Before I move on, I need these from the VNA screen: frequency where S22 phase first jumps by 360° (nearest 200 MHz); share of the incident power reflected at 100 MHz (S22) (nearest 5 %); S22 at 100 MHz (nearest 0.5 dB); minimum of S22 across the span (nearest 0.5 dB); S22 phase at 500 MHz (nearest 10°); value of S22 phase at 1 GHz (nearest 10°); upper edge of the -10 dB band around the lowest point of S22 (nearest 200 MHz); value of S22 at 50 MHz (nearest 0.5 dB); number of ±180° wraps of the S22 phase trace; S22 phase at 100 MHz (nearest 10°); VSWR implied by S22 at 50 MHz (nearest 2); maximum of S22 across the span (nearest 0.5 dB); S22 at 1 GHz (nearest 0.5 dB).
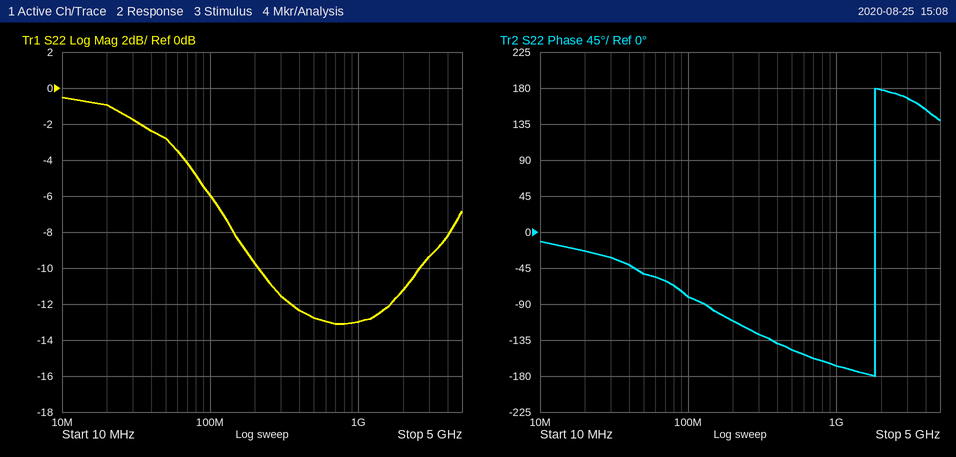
1.8 GHz
25 %
-6.0 dB
-13.0 dB
-150°
-170°
2.6 GHz
-3.0 dB
1
-80°
6
-0.5 dB
-13.0 dB
